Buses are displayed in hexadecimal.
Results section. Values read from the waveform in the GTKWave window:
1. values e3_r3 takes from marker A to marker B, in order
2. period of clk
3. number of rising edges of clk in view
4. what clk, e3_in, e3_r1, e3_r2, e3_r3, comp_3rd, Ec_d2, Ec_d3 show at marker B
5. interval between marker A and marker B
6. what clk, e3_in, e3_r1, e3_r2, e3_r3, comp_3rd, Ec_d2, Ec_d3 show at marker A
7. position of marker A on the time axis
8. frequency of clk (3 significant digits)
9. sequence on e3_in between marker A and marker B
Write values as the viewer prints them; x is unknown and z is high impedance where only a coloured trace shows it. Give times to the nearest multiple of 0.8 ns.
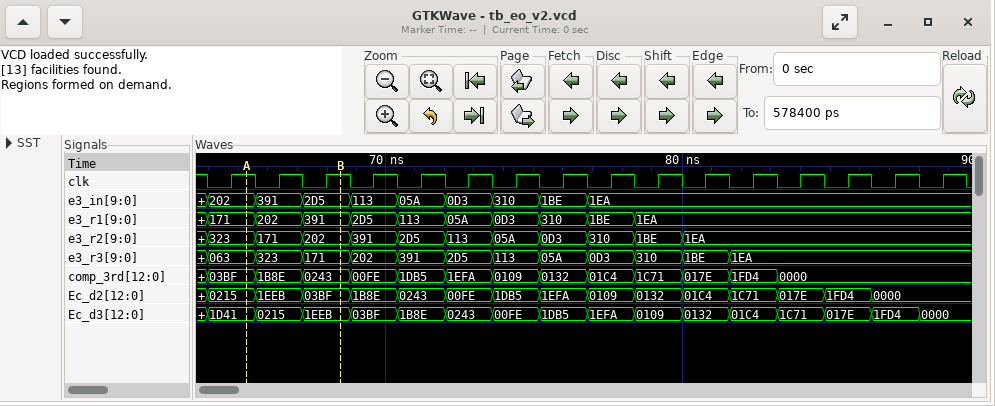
063, 323, 171
1.6 ns
16
clk=1, e3_in=2D5, e3_r1=391, e3_r2=202, e3_r3=171, comp_3rd=0243, Ec_d2=03BF, Ec_d3=1EEB
3.2 ns
clk=1, e3_in=202, e3_r1=171, e3_r2=323, e3_r3=063, comp_3rd=03BF, Ec_d2=0215, Ec_d3=1D41
65.6 ns
625 MHz
202, 391, 2D5
